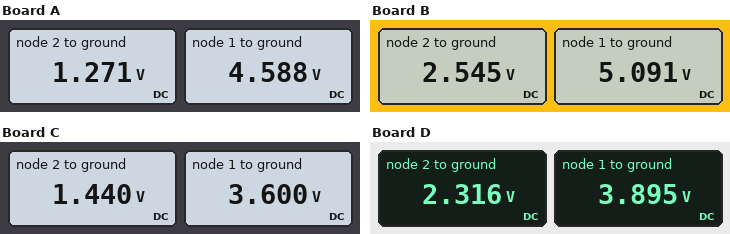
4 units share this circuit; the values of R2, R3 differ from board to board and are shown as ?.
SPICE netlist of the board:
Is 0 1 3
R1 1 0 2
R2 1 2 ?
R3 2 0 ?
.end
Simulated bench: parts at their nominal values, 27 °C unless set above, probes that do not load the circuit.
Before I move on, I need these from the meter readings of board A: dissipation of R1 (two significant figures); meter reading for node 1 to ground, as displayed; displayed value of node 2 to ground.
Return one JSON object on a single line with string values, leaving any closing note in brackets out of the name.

{"dissipation of R1": "11 W", "meter reading for node 1 to ground, as displayed": "4.588 V", "displayed value of node 2 to ground": "1.271 V"}
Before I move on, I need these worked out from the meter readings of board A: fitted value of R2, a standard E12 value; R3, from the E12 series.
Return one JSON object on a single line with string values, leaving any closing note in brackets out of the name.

{"fitted value of R2, a standard E12 value": "4.7 Ω", "R3, from the E12 series": "1.8 Ω"}
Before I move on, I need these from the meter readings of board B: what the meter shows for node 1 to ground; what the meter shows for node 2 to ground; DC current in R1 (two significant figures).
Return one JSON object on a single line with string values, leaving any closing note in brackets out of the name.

{"what the meter shows for node 1 to ground": "5.091 V", "what the meter shows for node 2 to ground": "2.545 V", "DC current in R1": "2.5 A"}
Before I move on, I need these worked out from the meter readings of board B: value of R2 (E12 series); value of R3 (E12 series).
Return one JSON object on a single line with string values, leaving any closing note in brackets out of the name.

{"value of R2": "5.6 Ω", "value of R3": "5.6 Ω"}
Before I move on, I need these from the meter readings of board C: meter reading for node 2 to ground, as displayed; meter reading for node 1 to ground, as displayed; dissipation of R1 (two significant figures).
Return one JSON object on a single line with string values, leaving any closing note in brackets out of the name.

{"meter reading for node 2 to ground, as displayed": "1.440 V", "meter reading for node 1 to ground, as displayed": "3.600 V", "dissipation of R1": "6.5 W"}
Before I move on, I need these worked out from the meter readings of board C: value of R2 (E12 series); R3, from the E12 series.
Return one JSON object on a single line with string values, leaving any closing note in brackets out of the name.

{"value of R2": "1.8 Ω", "R3, from the E12 series": "1.2 Ω"}
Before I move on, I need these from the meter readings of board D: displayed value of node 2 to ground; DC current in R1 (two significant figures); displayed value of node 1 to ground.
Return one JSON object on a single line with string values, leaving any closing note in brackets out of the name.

{"displayed value of node 2 to ground": "2.316 V", "DC current in R1": "1.9 A", "displayed value of node 1 to ground": "3.895 V"}
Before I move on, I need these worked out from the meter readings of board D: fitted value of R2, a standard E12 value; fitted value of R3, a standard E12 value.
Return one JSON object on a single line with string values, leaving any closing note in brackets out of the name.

{"fitted value of R2, a standard E12 value": "1.5 Ω", "fitted value of R3, a standard E12 value": "2.2 Ω"}
